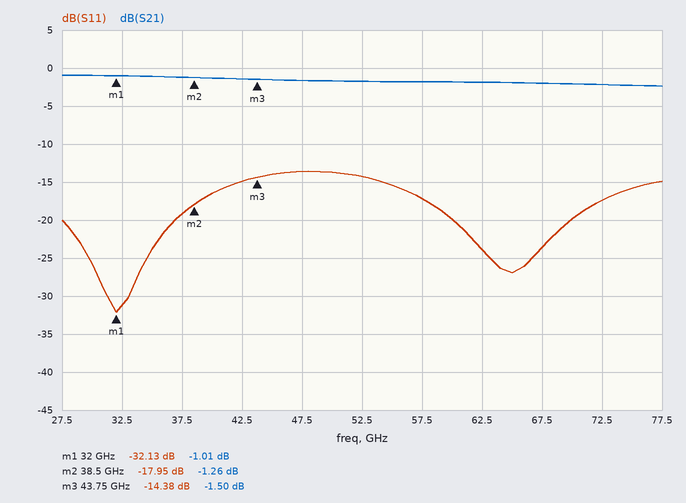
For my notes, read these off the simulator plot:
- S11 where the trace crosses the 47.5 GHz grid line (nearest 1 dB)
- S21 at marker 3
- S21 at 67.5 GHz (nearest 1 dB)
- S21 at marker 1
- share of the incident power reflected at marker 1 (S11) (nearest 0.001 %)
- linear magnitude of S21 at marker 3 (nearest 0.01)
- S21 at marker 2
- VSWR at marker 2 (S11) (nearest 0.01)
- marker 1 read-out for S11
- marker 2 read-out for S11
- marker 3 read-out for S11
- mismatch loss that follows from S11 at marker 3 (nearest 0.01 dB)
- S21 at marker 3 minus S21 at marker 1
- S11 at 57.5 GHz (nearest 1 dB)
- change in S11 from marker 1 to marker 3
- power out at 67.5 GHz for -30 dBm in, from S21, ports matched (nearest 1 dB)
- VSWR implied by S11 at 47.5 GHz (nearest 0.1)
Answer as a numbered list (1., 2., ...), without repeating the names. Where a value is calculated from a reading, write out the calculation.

1. -14 dB
2. -1.50 dB
3. -2 dB
4. -1.01 dB
5. 10^(-32.13/10) ≈ 0.061 %
6. 10^(-1.5/20) ≈ 0.84
7. -1.26 dB
8. (1 + 0.1266)/(1 − 0.1266) ≈ 1.29
9. -32.13 dB
10. -17.95 dB
11. -14.38 dB
12. −10 log10(1 − 10^(-14.38/10)) ≈ 0.16 dB
13. -1.5 − (-1.01) = -0.49 dB
14. -17 dB
15. -14.38 − (-32.13) = 17.75 dB
16. -30 dBm + (-2 dB) = -32 dBm
17. |Γ| = 10^(-14/20) = 0.1995; VSWR = (1 + 0.1995)/(1 − 0.1995) ≈ 1.5
